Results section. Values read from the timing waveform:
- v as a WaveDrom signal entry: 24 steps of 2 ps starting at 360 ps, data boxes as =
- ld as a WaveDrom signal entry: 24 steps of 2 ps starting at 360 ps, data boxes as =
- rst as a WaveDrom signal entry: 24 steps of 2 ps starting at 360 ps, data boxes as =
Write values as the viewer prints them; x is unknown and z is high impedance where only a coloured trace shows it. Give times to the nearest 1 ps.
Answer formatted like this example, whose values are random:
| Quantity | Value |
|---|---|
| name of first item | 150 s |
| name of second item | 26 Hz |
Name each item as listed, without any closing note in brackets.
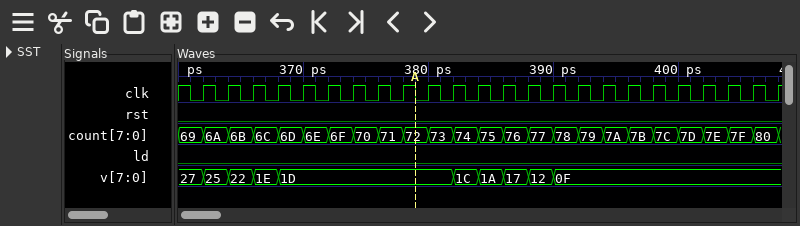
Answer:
| Quantity | Value |
|---|---|
| v as a WaveDrom signal entry: 24 steps of 2 ps starting at 360 ps, data boxes as = | {name: 'v', wave: '=====......=====........', data: '27 25 22 1E 1D 1C 1A 17 12 0F'} |
| ld as a WaveDrom signal entry: 24 steps of 2 ps starting at 360 ps, data boxes as = | {name: 'ld', wave: '0.......................'} |
| rst as a WaveDrom signal entry: 24 steps of 2 ps starting at 360 ps, data boxes as = | {name: 'rst', wave: '0.......................'} |
